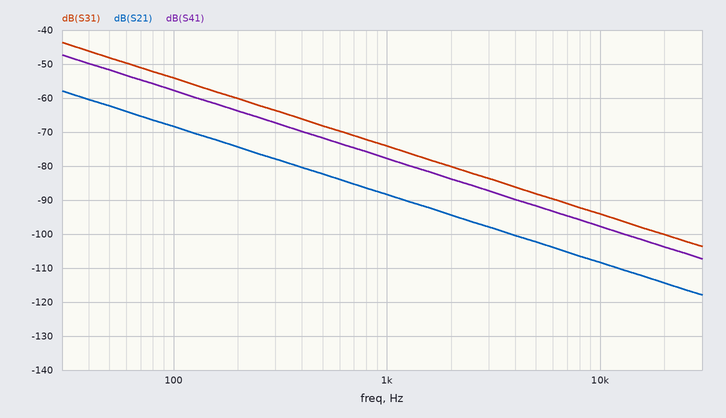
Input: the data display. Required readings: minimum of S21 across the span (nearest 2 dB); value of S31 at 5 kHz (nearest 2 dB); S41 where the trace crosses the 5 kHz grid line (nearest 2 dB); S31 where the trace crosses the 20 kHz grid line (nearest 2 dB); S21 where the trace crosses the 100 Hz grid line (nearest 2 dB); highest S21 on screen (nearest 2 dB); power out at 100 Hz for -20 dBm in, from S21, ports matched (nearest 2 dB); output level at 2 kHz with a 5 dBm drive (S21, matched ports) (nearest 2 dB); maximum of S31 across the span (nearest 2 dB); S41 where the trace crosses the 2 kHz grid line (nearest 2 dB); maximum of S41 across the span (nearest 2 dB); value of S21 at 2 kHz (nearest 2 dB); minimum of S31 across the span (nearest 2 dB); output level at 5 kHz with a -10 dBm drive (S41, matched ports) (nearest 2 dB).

-118 dB
-88 dB
-92 dB
-100 dB
-68 dB
-58 dB
-88 dBm
-90 dBm
-44 dB
-84 dB
-48 dB
-94 dB
-104 dB
-102 dBm
